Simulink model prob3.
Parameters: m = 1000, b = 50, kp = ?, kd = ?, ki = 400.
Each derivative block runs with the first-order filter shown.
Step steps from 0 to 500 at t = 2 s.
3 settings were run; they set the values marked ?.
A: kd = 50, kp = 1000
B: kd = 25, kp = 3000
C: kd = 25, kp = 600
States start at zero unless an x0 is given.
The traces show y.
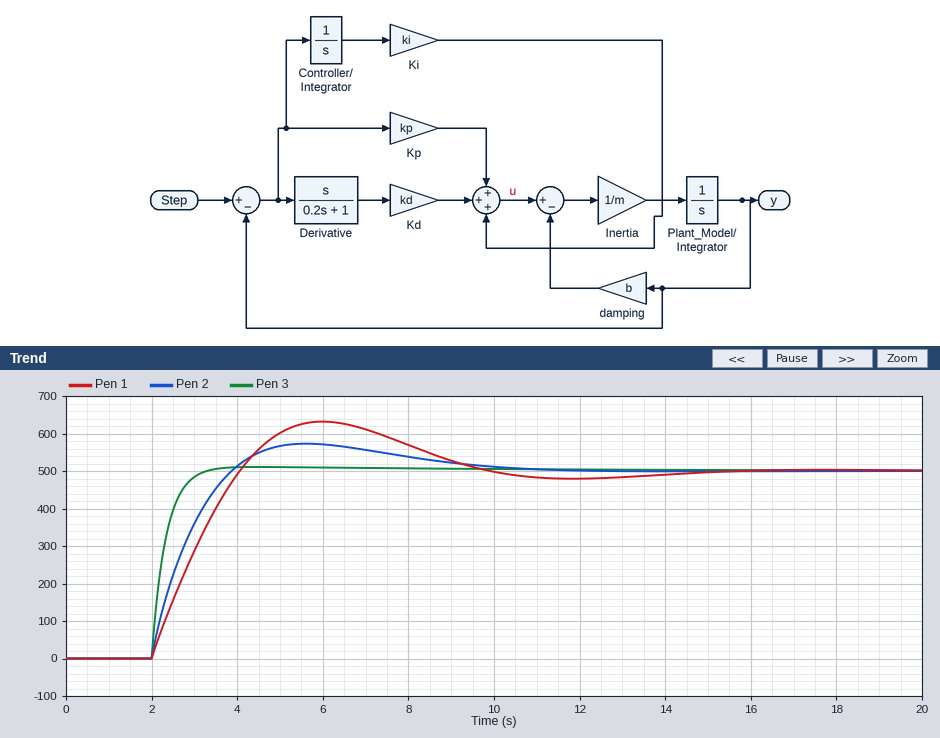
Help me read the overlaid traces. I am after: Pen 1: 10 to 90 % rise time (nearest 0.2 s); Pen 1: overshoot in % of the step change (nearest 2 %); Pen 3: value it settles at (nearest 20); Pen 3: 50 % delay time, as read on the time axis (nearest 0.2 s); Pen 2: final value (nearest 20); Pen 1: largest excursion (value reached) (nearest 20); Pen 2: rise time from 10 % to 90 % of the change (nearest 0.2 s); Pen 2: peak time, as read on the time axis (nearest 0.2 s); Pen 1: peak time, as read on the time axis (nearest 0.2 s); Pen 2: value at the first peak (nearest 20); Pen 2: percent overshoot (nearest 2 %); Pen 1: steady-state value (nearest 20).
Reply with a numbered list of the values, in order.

1. 1.6 s
2. 26 %
3. 500
4. 2.2 s
5. 500
6. 640
7. 1.4 s
8. 5.6 s
9. 6.0 s
10. 580
11. 14 %
12. 500
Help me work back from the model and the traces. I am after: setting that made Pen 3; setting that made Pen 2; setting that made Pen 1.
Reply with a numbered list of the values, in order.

1. B
2. A
3. C
